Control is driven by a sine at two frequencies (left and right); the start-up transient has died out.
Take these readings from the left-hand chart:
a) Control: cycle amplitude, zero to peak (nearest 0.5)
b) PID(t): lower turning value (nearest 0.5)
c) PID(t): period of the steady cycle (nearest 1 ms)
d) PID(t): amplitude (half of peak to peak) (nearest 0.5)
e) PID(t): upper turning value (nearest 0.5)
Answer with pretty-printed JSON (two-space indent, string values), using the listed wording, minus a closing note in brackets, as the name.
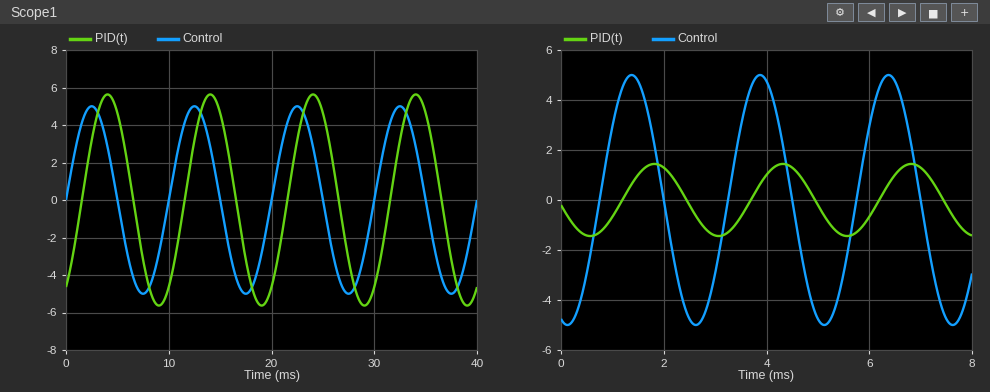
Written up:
{
  "Control: cycle amplitude, zero to peak": "5.0",
  "PID(t): lower turning value": "-5.5",
  "PID(t): period of the steady cycle": "10 ms",
  "PID(t): amplitude (half of peak to peak)": "5.5",
  "PID(t): upper turning value": "5.5"
}
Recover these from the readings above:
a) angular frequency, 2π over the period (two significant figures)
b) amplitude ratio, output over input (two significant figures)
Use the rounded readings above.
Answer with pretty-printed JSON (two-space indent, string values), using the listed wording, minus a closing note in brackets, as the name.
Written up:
{
  "angular frequency, 2π over the period": "0.63 rad/ms",
  "amplitude ratio, output over input": "1.1"
}
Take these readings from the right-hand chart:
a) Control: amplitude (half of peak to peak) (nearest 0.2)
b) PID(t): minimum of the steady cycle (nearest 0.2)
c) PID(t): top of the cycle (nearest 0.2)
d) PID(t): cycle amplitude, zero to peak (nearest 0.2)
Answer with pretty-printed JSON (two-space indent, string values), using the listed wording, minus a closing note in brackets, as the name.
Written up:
{
  "Control: amplitude (half of peak to peak)": "5.0",
  "PID(t): minimum of the steady cycle": "-1.4",
  "PID(t): top of the cycle": "1.4",
  "PID(t): cycle amplitude, zero to peak": "1.4"
}
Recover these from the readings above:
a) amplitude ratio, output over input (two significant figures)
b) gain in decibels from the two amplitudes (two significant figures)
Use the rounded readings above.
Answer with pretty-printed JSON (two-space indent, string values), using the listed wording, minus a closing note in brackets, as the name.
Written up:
{
  "amplitude ratio, output over input": "0.28",
  "gain in decibels from the two amplitudes": "-11 dB"
}
